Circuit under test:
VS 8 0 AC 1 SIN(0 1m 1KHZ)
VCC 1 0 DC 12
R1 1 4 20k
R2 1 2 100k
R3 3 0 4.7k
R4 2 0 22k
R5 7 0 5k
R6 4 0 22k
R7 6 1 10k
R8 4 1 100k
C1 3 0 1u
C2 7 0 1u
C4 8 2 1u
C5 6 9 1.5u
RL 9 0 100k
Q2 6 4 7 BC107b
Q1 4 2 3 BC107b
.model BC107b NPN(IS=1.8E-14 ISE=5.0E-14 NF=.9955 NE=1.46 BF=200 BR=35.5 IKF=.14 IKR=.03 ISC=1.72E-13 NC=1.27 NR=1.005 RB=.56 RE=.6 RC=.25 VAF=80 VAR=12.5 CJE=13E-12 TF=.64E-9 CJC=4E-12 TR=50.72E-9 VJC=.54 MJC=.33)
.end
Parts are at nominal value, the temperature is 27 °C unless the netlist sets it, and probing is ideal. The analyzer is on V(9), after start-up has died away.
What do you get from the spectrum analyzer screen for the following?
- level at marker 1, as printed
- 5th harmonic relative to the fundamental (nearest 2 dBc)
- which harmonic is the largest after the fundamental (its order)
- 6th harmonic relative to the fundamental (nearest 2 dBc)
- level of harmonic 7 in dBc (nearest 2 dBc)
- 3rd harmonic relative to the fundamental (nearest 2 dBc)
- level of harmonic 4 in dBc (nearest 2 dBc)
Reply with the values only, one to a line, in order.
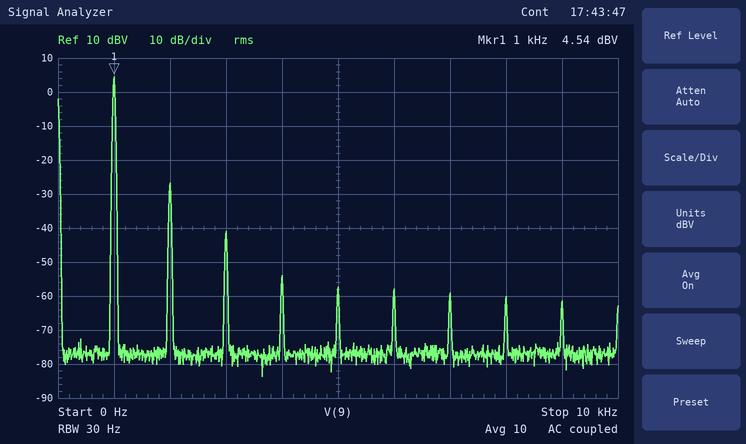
4.54 dBV
-62 dBc
2
-62 dBc
-64 dBc
-46 dBc
-58 dBc
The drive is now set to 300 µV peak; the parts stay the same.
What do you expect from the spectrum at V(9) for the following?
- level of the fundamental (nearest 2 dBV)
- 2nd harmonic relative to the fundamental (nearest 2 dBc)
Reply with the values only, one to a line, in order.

-6 dBV
-42 dBc
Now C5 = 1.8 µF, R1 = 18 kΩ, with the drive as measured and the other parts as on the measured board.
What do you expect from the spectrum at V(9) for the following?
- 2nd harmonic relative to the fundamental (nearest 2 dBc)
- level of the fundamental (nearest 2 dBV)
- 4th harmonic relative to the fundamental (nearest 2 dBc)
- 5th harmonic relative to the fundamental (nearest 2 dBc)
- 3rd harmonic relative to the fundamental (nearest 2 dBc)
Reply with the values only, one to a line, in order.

-12 dBc
2 dBV
-30 dBc
-28 dBc
-20 dBc
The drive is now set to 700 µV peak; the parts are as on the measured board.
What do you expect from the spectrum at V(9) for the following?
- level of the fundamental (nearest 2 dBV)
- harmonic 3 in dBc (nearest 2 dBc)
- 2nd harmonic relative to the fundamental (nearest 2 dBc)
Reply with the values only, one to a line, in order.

2 dBV
-54 dBc
-34 dBc
